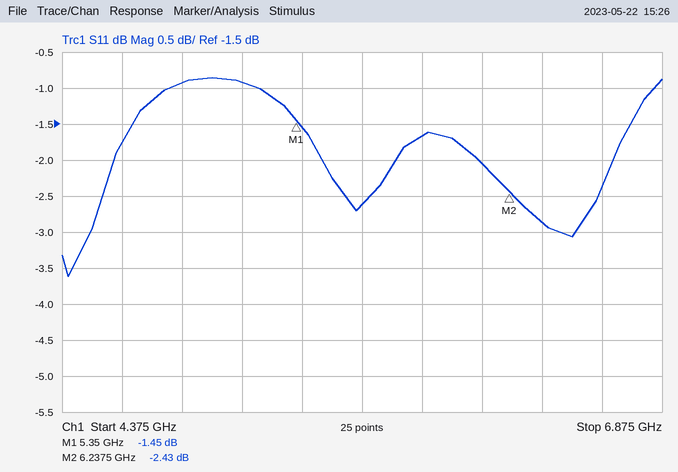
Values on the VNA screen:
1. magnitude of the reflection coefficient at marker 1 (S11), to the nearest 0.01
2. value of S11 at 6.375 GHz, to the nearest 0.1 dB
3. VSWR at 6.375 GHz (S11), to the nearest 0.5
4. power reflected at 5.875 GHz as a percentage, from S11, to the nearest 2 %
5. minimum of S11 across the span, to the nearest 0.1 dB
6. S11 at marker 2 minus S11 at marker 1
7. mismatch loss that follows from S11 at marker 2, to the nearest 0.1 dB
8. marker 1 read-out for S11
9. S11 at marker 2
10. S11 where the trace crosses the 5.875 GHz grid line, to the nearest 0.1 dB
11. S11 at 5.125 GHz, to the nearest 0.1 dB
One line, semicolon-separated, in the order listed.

0.85; -2.9 dB; 6.0; 68 %; -3.6 dB; -0.98 dB; 3.7 dB; -1.45 dB; -2.43 dB; -1.7 dB; -0.9 dB
